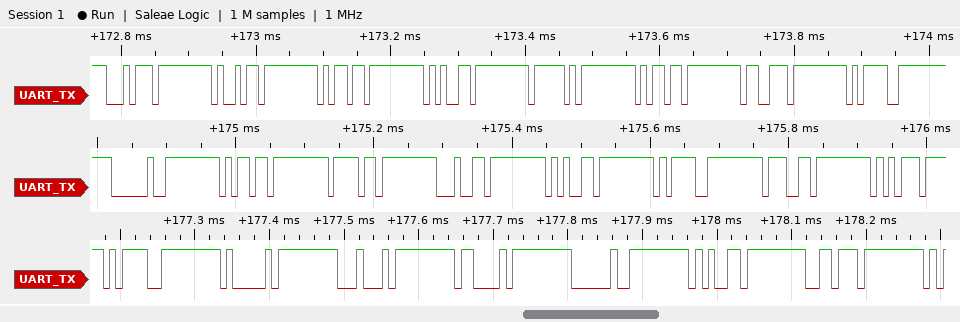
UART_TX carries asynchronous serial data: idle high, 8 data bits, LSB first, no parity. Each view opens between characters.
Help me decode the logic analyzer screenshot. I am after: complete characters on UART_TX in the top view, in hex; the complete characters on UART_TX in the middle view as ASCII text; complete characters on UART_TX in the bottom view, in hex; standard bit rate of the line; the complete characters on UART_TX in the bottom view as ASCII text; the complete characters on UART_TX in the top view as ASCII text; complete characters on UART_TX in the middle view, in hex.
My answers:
74, 69, 6D, 65, 5F, 6D, 73, 3D
" mode=gu"
3D, 41, 44, 43, 20, 65, 76
115200 baud
"=ADC ev"
"time_ms="
20, 6D, 6F, 64, 65, 3D, 67, 75
